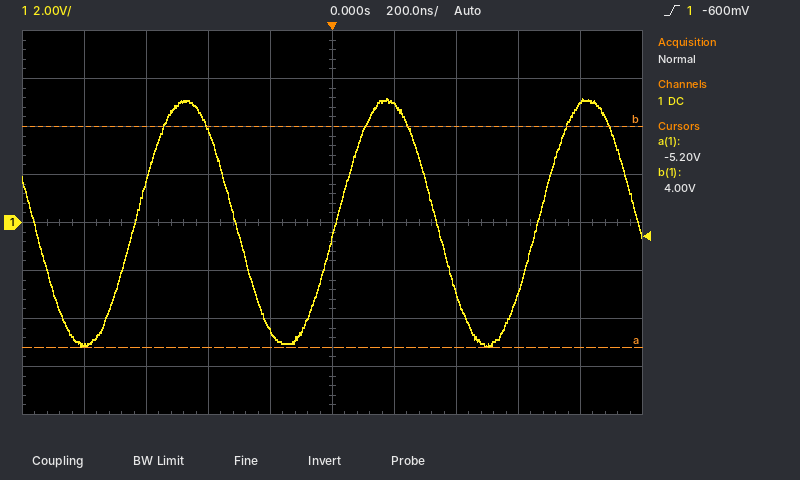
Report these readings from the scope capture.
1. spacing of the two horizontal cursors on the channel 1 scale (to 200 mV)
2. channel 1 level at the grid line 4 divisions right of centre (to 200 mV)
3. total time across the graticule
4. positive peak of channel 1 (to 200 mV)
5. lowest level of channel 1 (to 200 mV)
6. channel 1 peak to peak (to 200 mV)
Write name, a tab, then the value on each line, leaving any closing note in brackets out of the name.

spacing of the two horizontal cursors on the channel 1 scale	9.2 V
channel 1 level at the grid line 4 divisions right of centre	5.0 V
total time across the graticule	2 µs
positive peak of channel 1	5.2 V
lowest level of channel 1	-5.2 V
channel 1 peak to peak	10.4 V
